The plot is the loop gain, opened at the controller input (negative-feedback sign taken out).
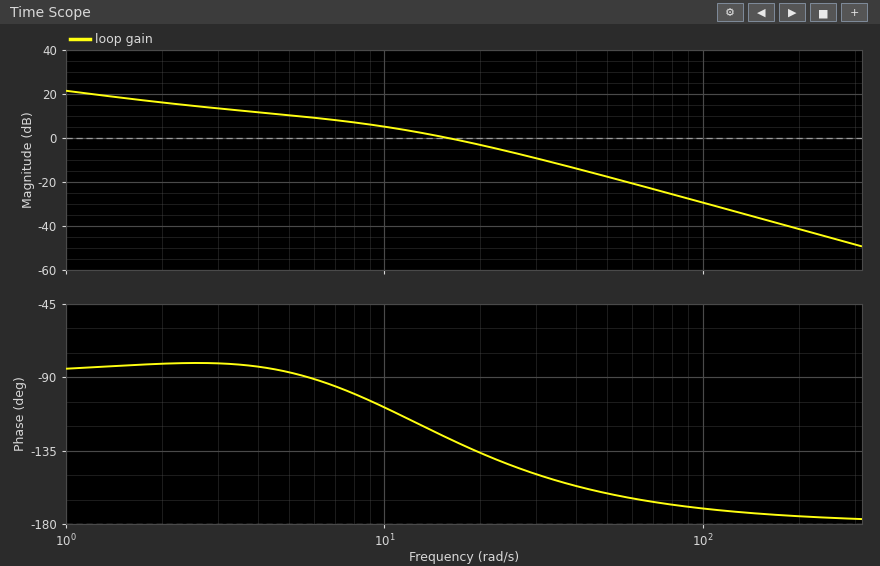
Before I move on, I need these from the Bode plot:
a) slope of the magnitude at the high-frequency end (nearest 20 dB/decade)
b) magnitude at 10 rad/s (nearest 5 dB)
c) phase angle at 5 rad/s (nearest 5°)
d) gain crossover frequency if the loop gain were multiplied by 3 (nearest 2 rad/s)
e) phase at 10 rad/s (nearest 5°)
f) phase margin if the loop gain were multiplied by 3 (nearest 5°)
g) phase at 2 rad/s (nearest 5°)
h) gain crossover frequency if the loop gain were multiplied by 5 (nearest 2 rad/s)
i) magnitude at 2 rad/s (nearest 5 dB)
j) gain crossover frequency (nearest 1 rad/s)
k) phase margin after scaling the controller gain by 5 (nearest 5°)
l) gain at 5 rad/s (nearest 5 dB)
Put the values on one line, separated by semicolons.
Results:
-40 dB/decade; 5 dB; -85°; 30 rad/s; -110°; 30°; -80°; 40 rad/s; 15 dB; 16 rad/s; 25°; 10 dB
